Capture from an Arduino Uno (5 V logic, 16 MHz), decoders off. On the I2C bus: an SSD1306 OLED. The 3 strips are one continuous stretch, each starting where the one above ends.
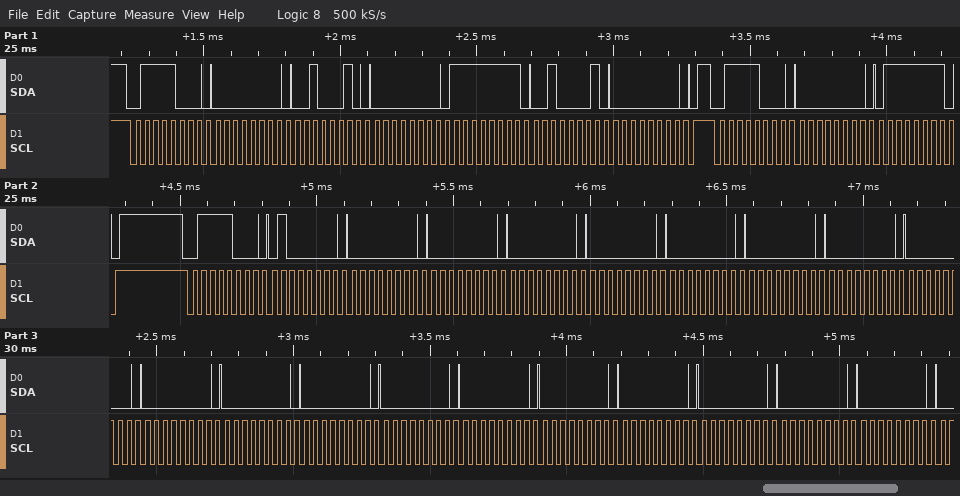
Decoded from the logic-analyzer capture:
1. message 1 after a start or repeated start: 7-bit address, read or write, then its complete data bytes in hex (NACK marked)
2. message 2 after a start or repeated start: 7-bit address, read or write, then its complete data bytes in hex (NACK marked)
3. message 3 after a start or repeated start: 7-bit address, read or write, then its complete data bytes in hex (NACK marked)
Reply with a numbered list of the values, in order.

1. 0x3C write: 00 22 00 FF 21 00
2. 0x3C write: 00 7F
3. 0x3C write: 40 00 00 00 00 00 00 00 00 00 00 00 00 00 00 00 00 00 00
